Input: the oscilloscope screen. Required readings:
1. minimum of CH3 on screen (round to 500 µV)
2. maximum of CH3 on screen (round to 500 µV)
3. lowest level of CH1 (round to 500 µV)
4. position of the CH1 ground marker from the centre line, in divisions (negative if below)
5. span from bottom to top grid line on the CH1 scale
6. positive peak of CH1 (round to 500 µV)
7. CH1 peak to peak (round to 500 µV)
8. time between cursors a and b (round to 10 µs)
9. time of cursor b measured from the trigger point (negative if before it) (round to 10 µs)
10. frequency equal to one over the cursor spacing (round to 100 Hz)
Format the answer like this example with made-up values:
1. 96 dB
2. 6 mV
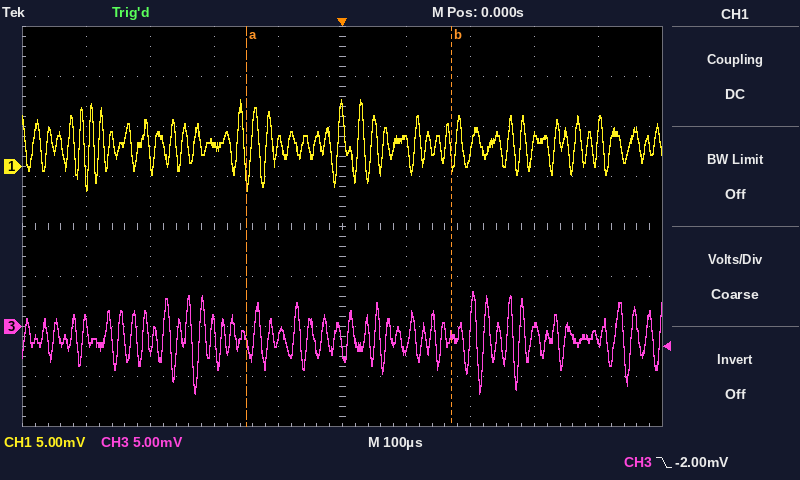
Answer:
1. -6.5 mV
2. 3.5 mV
3. -2.5 mV
4. +1.2 div
5. 40 mV
6. 6.5 mV
7. 9.0 mV
8. 320 µs
9. +170 µs
10. 3.1 kHz
